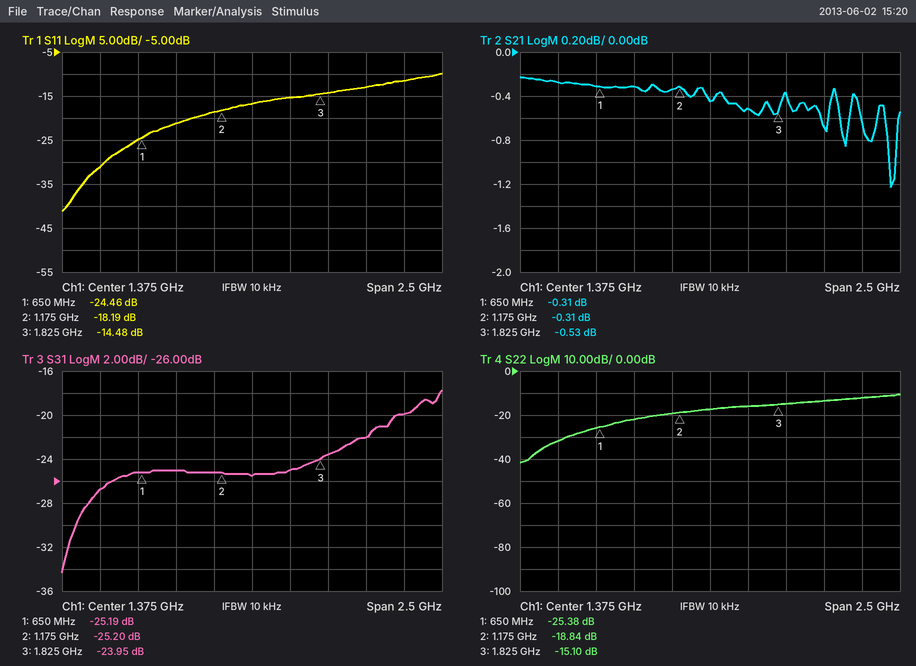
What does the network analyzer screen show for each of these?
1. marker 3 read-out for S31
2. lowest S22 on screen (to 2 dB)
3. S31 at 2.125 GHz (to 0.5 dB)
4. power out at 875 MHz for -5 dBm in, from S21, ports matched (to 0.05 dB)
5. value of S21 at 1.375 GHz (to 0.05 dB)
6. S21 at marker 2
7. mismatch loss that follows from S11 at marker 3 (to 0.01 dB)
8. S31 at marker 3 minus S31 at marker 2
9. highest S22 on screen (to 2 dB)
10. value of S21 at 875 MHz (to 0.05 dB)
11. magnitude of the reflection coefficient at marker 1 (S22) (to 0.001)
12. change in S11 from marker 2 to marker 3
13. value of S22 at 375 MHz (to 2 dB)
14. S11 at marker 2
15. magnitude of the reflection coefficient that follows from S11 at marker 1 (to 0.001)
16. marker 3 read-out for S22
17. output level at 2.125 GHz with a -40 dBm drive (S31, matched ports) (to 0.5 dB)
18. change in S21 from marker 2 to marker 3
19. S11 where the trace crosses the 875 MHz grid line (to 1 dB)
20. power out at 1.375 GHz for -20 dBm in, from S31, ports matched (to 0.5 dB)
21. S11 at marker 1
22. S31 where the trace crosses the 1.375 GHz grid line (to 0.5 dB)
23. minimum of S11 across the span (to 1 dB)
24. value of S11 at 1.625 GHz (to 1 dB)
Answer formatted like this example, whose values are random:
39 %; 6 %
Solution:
-23.95 dB; -42 dB; -22.0 dB; -5.30 dBm; -0.45 dB; -0.31 dB; 0.16 dB; 1.25 dB; -10 dB; -0.30 dB; 0.054; 3.71 dB; -32 dB; -18.19 dB; 0.060; -15.10 dB; -62.0 dBm; -0.22 dB; -21 dB; -45.5 dBm; -24.46 dB; -25.5 dB; -41 dB; -15 dB
